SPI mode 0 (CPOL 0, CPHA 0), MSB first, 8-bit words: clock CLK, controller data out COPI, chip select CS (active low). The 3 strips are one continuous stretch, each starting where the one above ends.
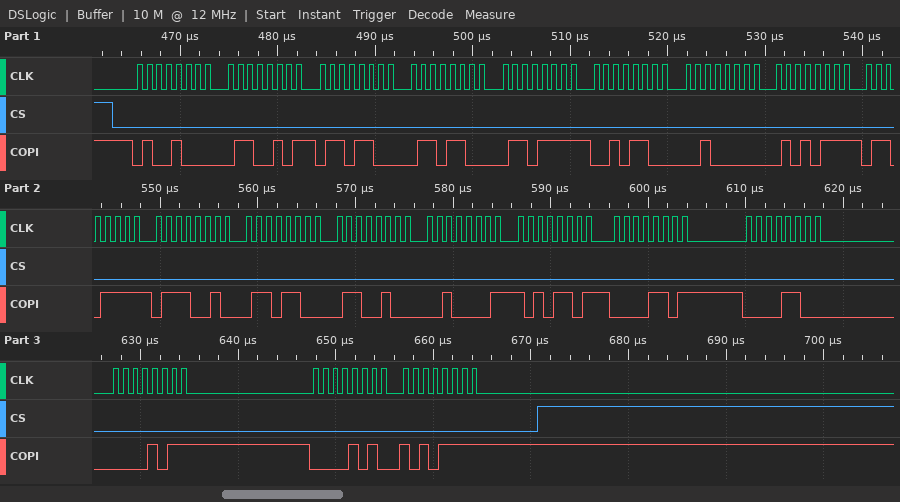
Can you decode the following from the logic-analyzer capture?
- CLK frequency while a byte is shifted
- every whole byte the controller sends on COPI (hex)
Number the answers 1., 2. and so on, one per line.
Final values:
1. 1 MHz
2. 0x48 0x65 0x6C 0x6C 0x6F 0x2C 0x20 0x57 0x6F 0x72 0x6C 0x64 0x21 0xAD 0x0D 0x0C 0x0B 0x0A 0xAF
